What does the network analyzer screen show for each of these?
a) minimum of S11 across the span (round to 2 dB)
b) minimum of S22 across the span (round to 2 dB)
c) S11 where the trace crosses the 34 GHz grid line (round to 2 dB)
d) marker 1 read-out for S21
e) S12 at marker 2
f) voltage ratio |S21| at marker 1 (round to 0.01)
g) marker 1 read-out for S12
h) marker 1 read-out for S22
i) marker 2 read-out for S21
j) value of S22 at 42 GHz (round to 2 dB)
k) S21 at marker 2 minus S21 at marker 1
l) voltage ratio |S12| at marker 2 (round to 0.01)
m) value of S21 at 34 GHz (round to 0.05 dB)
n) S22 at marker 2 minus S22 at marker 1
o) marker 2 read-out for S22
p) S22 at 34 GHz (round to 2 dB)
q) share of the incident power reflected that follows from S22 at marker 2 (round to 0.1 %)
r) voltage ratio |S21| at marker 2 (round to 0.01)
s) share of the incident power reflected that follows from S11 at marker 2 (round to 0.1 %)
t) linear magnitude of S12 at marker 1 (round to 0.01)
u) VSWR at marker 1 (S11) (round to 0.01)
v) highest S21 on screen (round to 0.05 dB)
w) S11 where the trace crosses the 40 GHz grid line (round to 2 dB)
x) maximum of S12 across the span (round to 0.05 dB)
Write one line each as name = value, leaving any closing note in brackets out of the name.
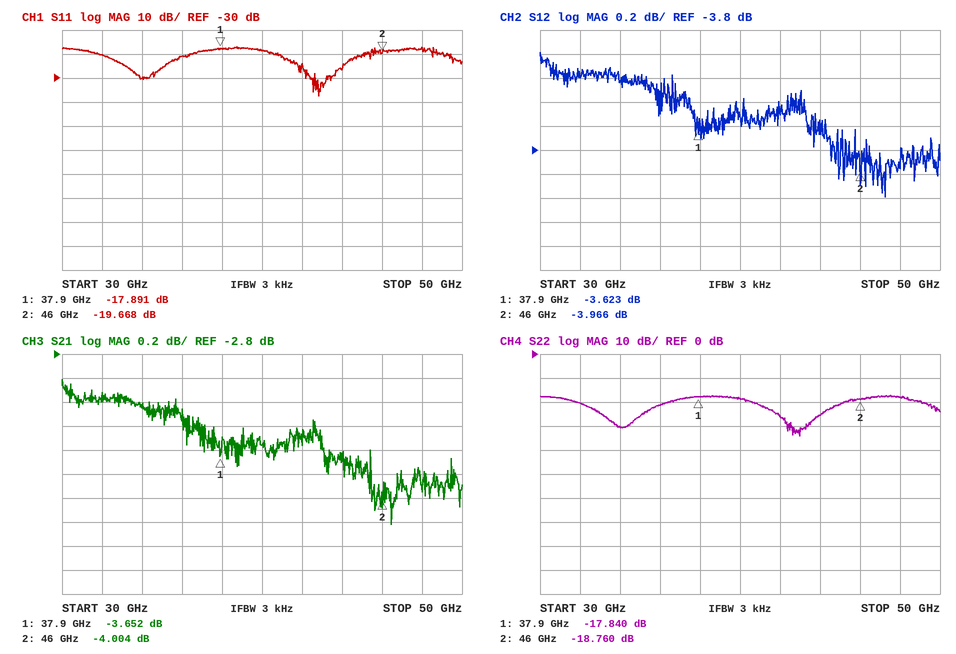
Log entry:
minimum of S11 across the span = -38 dB
minimum of S22 across the span = -34 dB
S11 where the trace crosses the 34 GHz grid line = -30 dB
marker 1 read-out for S21 = -3.652 dB
S12 at marker 2 = -3.966 dB
voltage ratio |S21| at marker 1 = 0.66
marker 1 read-out for S12 = -3.623 dB
marker 1 read-out for S22 = -17.840 dB
marker 2 read-out for S21 = -4.004 dB
value of S22 at 42 GHz = -26 dB
S21 at marker 2 minus S21 at marker 1 = -0.352 dB
voltage ratio |S12| at marker 2 = 0.63
value of S21 at 34 GHz = -3.25 dB
S22 at marker 2 minus S22 at marker 1 = -0.920 dB
marker 2 read-out for S22 = -18.760 dB
S22 at 34 GHz = -30 dB
share of the incident power reflected that follows from S22 at marker 2 = 1.3 %
voltage ratio |S21| at marker 2 = 0.63
share of the incident power reflected that follows from S11 at marker 2 = 1.1 %
linear magnitude of S12 at marker 1 = 0.66
VSWR at marker 1 (S11) = 1.29
highest S21 on screen = -3.00 dB
S11 where the trace crosses the 40 GHz grid line = -18 dB
maximum of S12 across the span = -3.00 dB
